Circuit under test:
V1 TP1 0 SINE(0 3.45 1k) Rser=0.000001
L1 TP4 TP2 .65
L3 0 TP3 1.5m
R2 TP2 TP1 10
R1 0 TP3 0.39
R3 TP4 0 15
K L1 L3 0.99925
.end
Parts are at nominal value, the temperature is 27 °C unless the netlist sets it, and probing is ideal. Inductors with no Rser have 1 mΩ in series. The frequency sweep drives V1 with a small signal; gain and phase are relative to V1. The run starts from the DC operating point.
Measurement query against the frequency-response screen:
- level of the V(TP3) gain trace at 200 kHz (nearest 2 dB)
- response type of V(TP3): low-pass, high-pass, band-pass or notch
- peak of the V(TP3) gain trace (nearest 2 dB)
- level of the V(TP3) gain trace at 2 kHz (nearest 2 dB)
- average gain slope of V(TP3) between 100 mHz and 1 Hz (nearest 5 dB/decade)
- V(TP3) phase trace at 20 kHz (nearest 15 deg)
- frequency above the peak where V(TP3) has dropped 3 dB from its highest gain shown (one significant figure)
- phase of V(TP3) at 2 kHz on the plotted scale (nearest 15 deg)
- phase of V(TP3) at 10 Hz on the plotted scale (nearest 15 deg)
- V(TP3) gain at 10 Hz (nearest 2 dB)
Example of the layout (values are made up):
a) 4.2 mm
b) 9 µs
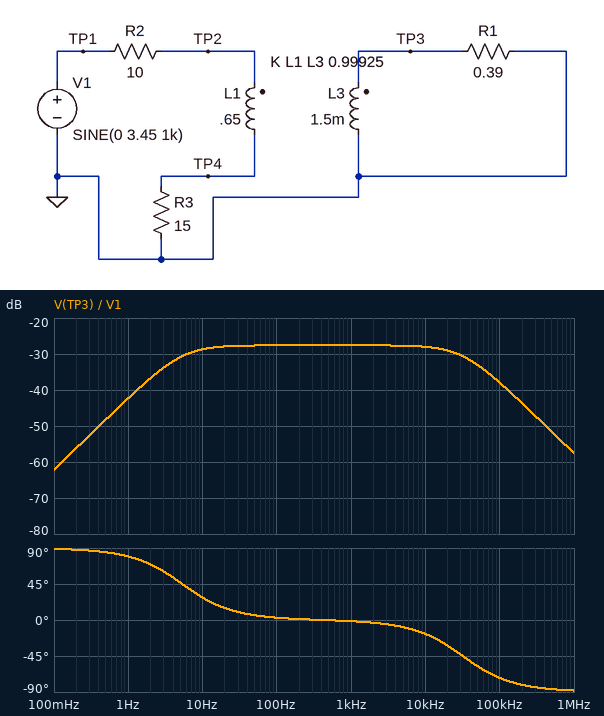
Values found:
a) -44 dB
b) band-pass
c) -28 dB
d) -28 dB
e) 20 dB/decade
f) -30 deg
g) 30 kHz
h) 0 deg
i) 30 deg
j) -28 dB
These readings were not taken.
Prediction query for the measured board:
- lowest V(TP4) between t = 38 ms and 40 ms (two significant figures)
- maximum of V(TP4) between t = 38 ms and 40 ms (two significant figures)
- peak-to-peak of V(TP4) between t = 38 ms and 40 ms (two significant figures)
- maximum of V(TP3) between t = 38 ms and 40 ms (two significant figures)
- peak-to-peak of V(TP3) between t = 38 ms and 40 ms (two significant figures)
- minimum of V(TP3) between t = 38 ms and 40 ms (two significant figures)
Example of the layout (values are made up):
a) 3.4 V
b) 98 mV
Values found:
a) -260 mV
b) 270 mV
c) 530 mV
d) 140 mV
e) 290 mV
f) -140 mV
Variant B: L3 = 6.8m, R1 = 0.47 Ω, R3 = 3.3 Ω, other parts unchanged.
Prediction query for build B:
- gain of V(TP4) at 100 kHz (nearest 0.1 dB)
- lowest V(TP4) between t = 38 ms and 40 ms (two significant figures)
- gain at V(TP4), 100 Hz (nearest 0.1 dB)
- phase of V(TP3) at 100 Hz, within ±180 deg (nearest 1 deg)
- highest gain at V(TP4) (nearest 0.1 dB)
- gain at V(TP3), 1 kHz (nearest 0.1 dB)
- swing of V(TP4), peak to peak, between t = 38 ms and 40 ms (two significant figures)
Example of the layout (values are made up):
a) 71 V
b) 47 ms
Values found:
a) -45.4 dB
b) -190 mV
c) -24.9 dB
d) 1 deg
e) -12.1 dB
f) -22.1 dB
g) 390 mV
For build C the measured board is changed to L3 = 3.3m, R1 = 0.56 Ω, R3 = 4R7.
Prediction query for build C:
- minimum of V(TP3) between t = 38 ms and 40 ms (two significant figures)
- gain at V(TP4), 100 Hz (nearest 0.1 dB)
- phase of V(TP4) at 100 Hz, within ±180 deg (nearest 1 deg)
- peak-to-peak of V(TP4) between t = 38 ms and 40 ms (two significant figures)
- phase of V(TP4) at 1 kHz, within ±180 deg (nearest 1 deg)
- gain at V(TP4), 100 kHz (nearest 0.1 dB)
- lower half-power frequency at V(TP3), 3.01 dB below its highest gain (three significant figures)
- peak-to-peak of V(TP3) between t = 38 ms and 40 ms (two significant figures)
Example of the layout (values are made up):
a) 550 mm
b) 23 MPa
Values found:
a) -220 mV
b) -28.2 dB
c) -14 deg
d) 260 mV
e) -4 deg
f) -42.5 dB
g) 3.18 Hz
h) 430 mV
